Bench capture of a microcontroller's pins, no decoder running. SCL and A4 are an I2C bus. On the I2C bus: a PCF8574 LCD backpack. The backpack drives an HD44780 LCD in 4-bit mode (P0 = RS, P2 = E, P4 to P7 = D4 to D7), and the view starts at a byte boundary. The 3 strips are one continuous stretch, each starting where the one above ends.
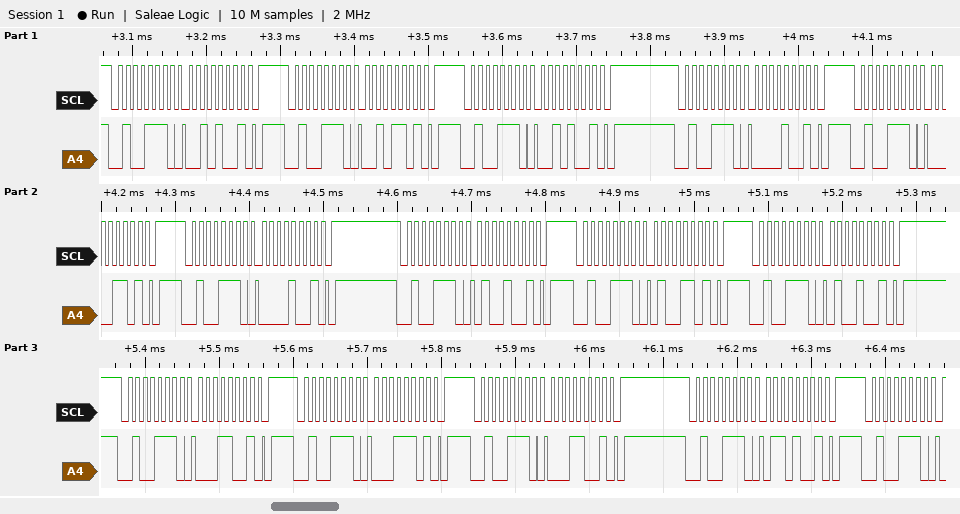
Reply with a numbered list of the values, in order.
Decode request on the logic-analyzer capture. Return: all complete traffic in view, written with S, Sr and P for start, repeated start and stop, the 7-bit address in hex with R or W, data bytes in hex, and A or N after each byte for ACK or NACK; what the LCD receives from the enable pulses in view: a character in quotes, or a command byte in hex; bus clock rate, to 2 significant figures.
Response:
1. S 27W A 29 A P S 27W A 2D A P S 27W A 29 A P S 27W A 09 A P S 27W A 0D A P S 27W A 09 A P S 27W A 49 A P S 27W A 4D A P S 27W A 49 A P S 27W A 19 A P S 27W A 1D A P S 27W A 19 A P S 27W A 69 A P S 27W A
2. ' ' 'A'
3. 100 kHz
